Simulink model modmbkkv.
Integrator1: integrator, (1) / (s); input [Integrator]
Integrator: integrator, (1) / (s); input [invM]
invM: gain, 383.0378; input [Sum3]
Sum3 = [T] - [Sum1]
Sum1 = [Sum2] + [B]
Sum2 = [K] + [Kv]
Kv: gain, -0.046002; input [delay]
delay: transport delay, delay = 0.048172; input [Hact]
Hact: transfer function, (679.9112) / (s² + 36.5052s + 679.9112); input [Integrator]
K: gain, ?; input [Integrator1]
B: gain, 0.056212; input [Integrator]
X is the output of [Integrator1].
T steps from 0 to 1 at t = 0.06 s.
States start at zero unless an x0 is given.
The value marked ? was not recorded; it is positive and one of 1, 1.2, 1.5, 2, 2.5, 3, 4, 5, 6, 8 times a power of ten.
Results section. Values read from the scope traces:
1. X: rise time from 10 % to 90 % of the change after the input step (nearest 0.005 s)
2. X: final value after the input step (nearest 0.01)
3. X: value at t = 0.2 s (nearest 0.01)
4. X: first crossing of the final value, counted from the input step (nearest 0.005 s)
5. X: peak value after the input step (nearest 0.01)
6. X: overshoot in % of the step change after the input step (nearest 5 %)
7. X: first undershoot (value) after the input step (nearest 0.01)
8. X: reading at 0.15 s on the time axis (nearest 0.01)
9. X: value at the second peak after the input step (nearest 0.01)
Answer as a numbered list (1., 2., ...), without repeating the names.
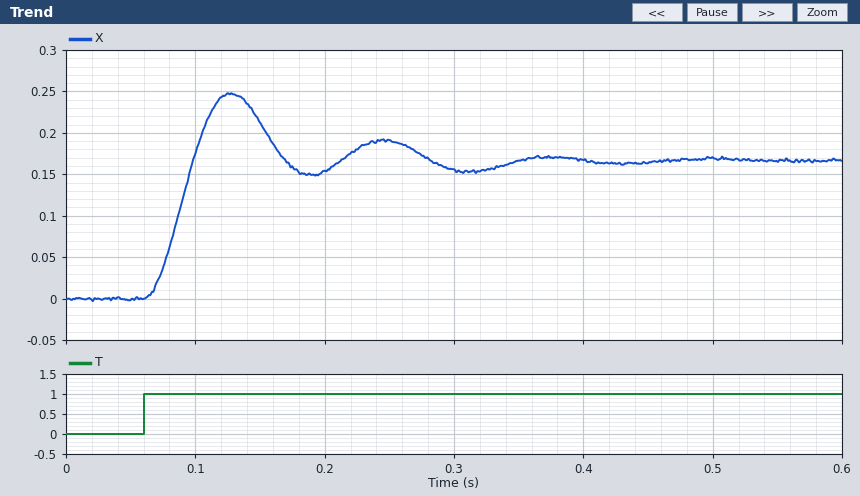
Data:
1. 0.025 s
2. 0.17
3. 0.15
4. 0.040 s
5. 0.25
6. 50 %
7. 0.15
8. 0.21
9. 0.19
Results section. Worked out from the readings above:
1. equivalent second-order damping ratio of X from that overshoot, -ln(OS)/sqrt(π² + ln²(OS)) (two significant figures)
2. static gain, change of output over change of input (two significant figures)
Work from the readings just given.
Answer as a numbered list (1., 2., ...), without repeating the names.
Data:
1. 0.22
2. 0.17
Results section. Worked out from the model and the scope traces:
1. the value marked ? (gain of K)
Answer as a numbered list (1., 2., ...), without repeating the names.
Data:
1. 6
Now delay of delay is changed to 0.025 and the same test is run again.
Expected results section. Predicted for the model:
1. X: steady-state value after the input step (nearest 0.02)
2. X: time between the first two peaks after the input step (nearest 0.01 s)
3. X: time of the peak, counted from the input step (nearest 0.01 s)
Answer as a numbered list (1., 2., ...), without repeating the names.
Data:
1. 0.16
2. 0.12 s
3. 0.07 s
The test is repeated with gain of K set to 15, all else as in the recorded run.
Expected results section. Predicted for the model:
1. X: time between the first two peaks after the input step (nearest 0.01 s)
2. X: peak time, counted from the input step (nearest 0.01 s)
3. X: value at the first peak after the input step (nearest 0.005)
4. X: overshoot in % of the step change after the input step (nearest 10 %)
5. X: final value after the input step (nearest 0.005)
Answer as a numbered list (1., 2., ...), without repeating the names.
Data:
1. 0.08 s
2. 0.04 s
3. 0.110
4. 60 %
5. 0.065
